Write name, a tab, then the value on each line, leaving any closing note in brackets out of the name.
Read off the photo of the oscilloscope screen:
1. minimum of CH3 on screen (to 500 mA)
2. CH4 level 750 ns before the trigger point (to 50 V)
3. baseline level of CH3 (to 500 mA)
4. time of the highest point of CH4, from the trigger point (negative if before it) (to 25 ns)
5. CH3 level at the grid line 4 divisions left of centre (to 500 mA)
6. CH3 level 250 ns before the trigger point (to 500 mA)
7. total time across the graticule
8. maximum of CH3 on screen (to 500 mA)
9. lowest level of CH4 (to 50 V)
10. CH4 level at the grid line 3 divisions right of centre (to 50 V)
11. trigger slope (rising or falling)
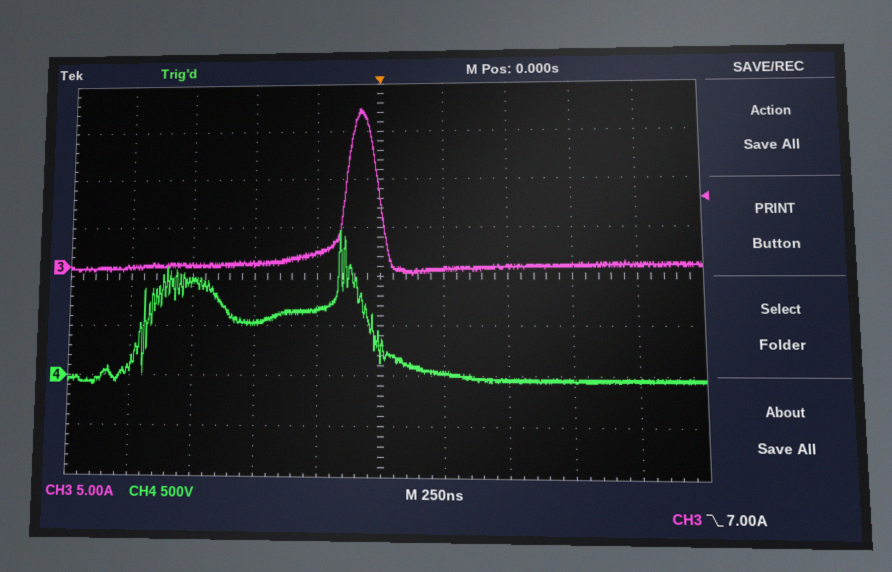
minimum of CH3 on screen	-1.0 A
CH4 level 750 ns before the trigger point	950 V
baseline level of CH3	0.0 A
time of the highest point of CH4, from the trigger point (negative if before it)	-150 ns
CH3 level at the grid line 4 divisions left of centre	0.0 A
CH3 level 250 ns before the trigger point	1.5 A
total time across the graticule	2.5 µs
maximum of CH3 on screen	16.5 A
lowest level of CH4	-100 V
CH4 level at the grid line 3 divisions right of centre	-50 V
trigger slope	falling
